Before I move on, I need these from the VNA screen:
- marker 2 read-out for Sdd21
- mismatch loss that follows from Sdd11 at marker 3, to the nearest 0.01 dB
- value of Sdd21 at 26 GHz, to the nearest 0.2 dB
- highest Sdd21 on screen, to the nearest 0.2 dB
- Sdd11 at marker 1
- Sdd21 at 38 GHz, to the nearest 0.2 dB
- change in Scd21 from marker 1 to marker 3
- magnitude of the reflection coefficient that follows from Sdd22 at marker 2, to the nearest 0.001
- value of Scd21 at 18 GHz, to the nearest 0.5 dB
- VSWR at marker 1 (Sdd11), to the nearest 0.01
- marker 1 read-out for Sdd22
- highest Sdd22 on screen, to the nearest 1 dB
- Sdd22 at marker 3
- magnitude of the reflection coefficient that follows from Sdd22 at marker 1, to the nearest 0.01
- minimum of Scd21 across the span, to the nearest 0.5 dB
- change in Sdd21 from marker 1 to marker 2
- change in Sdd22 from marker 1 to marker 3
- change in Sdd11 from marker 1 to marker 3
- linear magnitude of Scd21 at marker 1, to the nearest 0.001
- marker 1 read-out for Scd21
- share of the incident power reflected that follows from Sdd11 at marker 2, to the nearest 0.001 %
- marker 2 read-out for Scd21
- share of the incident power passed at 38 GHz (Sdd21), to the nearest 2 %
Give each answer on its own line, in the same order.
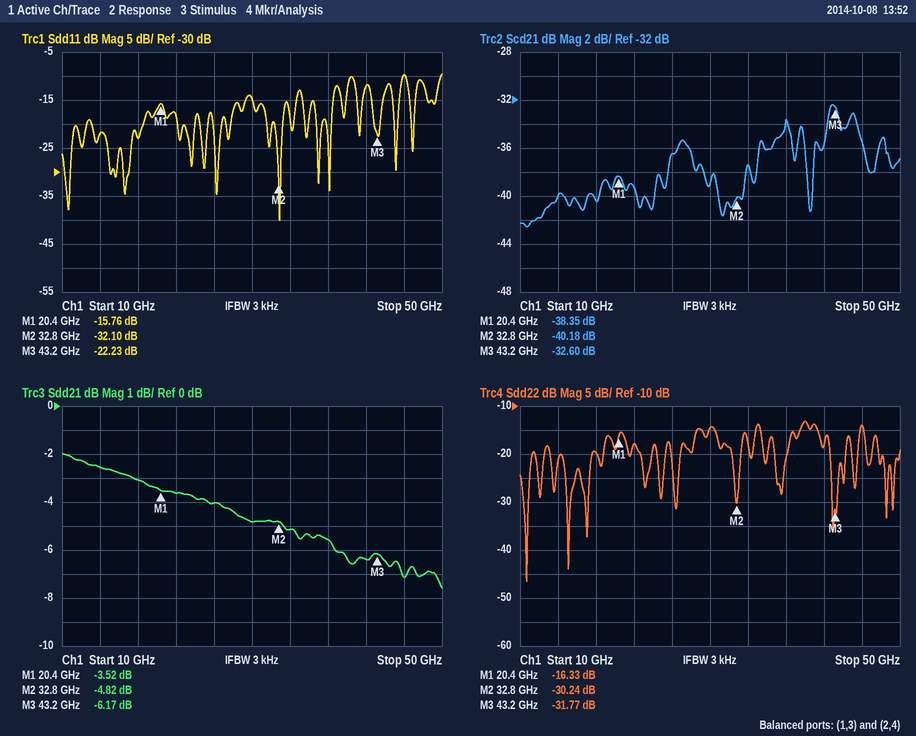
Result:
-4.82 dB
0.03 dB
-4.0 dB
-2.0 dB
-15.76 dB
-5.6 dB
5.75 dB
0.031
-40.5 dB
1.39
-16.33 dB
-13 dB
-31.77 dB
0.15
-42.5 dB
-1.30 dB
-15.44 dB
-6.47 dB
0.012
-38.35 dB
0.062 %
-40.18 dB
28 %
